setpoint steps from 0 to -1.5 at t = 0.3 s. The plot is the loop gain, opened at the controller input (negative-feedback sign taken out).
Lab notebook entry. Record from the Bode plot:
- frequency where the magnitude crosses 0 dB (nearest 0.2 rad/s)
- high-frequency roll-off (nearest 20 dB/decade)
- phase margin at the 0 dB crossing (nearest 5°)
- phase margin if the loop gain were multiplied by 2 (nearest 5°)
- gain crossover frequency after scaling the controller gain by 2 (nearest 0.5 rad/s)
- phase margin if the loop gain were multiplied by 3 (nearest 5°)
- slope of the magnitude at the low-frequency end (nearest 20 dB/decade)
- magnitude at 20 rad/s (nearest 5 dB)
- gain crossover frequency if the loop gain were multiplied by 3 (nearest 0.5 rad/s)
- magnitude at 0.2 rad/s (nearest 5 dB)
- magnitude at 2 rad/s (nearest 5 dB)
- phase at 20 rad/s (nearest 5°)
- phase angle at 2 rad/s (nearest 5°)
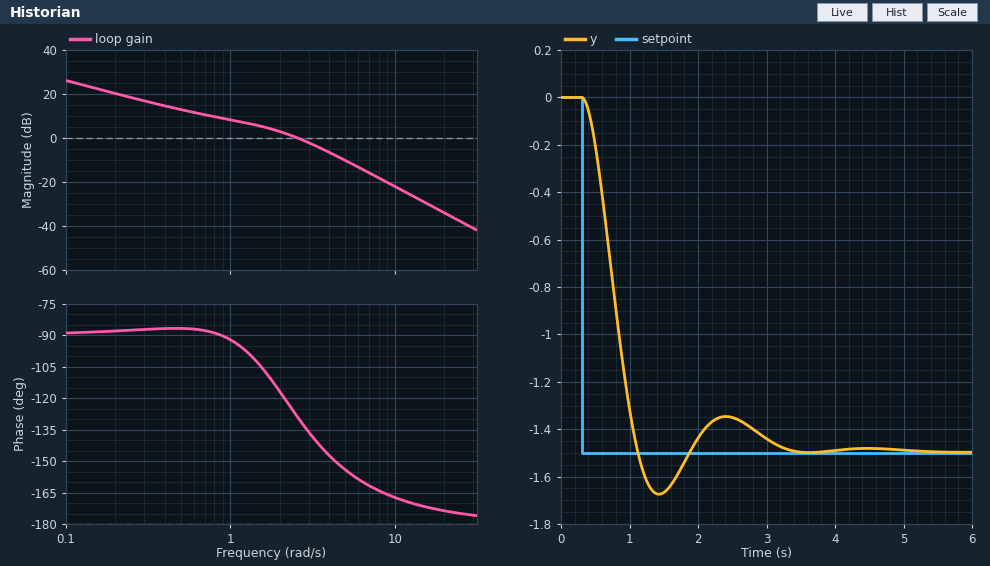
2.6 rad/s
-40 dB/decade
50°
35°
4.0 rad/s
25°
-20 dB/decade
-35 dB
5.0 rad/s
20 dB
5 dB
-175°
-115°
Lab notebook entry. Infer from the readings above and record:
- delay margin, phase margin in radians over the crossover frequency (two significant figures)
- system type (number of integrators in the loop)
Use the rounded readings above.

0.34 s
1
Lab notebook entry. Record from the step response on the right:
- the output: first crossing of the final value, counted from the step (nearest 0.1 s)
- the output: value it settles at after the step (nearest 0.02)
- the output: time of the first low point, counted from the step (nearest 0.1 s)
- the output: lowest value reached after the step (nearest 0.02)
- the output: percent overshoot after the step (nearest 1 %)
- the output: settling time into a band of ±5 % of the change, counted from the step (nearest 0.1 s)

0.8 s
-1.50
1.1 s
-1.68
12 %
2.6 s
